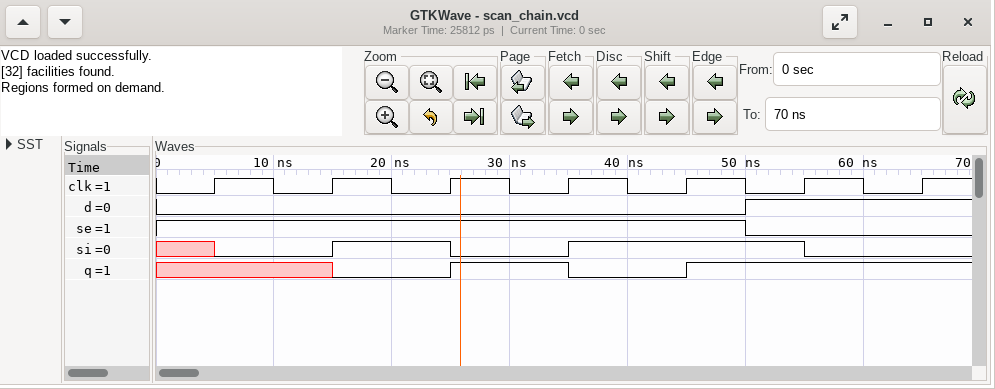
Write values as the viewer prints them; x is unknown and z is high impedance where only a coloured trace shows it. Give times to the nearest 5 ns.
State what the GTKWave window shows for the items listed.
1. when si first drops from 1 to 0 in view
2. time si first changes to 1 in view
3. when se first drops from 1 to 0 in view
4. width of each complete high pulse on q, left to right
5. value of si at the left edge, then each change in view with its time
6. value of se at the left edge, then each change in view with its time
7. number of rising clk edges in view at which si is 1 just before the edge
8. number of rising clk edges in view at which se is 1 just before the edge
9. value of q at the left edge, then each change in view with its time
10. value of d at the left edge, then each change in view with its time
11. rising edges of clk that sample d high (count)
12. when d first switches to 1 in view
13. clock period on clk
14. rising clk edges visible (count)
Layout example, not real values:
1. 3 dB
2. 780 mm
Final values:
1. 25 ns
2. 15 ns
3. 50 ns
4. 10 ns
5. x, 0 at 5 ns, 1 at 15 ns, 0 at 25 ns, 1 at 35 ns, 0 at 55 ns
6. 1, 0 at 50 ns
7. 3
8. 5
9. x, 0 at 15 ns, 1 at 25 ns, 0 at 35 ns, 1 at 45 ns
10. 0, 1 at 50 ns
11. 2
12. 50 ns
13. 10 ns
14. 7
